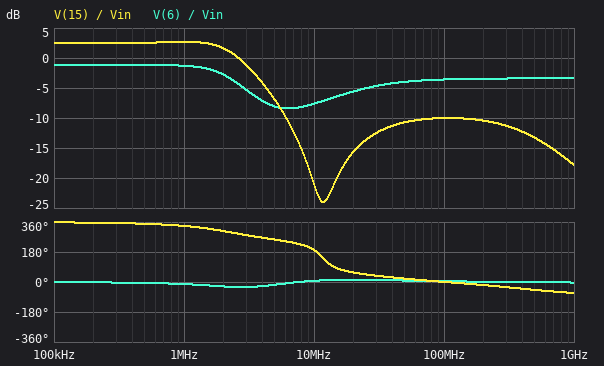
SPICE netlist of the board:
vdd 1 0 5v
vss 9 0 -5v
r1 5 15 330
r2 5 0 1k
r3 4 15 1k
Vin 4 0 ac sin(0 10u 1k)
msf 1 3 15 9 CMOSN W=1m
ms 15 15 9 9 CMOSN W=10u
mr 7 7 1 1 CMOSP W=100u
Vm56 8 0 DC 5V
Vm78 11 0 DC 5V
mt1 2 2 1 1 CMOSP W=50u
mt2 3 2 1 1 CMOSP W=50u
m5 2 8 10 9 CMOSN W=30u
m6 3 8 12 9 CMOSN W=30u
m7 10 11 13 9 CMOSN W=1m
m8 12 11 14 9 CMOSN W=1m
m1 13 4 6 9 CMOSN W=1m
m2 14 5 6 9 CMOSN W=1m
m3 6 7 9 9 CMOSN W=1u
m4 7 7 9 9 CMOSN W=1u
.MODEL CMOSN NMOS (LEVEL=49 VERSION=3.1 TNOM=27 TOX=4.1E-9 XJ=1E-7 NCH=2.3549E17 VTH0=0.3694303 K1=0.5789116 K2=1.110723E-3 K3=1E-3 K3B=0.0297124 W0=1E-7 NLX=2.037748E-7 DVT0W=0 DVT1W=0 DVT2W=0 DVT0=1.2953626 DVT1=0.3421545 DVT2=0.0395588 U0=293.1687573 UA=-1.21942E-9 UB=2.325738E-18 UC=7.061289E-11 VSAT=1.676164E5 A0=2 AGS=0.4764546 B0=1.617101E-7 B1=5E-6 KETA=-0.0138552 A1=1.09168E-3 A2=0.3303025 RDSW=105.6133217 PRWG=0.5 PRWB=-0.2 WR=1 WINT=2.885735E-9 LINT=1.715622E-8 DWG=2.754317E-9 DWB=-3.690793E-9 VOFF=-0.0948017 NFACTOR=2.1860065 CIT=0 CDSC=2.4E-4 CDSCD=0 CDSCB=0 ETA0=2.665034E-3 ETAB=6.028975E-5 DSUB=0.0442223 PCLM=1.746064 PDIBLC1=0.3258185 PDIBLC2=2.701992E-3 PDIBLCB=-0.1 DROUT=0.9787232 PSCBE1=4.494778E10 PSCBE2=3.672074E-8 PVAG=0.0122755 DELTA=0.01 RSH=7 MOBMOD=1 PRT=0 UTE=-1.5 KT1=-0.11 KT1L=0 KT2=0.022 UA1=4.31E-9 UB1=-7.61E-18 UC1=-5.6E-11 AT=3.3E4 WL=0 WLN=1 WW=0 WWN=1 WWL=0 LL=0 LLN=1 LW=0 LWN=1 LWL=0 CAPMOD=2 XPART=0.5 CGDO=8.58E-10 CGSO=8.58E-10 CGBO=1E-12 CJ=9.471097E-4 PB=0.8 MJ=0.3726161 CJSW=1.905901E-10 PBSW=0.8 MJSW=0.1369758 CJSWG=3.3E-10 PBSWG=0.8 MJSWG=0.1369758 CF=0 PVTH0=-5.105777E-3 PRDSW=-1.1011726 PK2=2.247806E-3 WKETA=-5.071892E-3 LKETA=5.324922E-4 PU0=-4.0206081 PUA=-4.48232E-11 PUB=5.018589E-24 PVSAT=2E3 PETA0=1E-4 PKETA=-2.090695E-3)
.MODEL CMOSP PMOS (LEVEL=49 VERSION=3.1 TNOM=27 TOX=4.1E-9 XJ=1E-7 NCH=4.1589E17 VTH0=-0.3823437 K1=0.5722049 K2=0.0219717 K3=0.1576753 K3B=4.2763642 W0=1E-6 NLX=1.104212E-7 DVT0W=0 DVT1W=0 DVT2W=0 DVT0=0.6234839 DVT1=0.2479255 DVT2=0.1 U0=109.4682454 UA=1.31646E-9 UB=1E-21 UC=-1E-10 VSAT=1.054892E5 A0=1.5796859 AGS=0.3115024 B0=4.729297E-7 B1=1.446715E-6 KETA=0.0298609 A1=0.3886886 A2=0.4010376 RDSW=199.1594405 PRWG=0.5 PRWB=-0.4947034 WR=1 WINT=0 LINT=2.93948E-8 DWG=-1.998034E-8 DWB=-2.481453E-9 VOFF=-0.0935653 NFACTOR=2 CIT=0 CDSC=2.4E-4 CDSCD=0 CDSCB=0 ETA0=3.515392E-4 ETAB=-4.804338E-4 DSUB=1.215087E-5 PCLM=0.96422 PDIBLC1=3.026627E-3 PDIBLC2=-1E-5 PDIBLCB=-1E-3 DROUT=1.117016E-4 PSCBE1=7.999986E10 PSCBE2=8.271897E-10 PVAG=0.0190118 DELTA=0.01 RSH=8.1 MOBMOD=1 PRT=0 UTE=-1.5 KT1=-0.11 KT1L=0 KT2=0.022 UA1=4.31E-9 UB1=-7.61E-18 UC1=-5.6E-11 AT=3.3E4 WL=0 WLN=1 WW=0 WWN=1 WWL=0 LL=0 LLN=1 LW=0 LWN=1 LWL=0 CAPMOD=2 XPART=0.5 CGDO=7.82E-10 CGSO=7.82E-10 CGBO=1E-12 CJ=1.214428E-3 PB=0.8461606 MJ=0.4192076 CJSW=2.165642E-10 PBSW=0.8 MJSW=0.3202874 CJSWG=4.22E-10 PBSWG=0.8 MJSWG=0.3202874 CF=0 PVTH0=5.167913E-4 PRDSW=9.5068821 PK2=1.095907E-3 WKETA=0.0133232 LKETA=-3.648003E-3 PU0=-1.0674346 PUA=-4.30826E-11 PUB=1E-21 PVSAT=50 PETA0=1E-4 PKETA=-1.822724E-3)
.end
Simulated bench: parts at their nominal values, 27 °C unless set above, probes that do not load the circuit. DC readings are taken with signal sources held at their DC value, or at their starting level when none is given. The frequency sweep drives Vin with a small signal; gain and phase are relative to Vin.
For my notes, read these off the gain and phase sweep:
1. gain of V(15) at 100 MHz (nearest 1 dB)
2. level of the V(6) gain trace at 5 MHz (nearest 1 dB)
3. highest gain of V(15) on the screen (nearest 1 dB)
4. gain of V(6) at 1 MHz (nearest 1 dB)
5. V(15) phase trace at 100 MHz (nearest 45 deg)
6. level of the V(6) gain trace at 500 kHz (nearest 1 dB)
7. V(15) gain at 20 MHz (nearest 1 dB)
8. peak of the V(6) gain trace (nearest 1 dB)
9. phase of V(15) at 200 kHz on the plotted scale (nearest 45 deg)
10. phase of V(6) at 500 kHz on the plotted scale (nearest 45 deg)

-10 dB
-8 dB
3 dB
-1 dB
0 deg
-1 dB
-16 dB
-1 dB
360 deg
0 deg
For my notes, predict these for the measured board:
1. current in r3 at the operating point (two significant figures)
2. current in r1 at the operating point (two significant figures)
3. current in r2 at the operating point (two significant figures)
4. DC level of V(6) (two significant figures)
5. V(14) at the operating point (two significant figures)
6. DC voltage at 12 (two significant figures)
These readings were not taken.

6.3 µA
4.7 µA
4.7 µA
-1.1 V
1.5 V
1.5 V
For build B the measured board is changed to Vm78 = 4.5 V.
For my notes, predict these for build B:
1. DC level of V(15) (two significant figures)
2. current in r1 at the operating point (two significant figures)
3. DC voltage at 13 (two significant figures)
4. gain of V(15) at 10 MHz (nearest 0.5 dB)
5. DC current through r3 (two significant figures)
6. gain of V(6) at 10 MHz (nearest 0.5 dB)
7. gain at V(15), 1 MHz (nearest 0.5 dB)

5.9 mV
4.4 µA
2.9 V
-4.0 dB
5.9 µA
-12.5 dB
2.0 dB
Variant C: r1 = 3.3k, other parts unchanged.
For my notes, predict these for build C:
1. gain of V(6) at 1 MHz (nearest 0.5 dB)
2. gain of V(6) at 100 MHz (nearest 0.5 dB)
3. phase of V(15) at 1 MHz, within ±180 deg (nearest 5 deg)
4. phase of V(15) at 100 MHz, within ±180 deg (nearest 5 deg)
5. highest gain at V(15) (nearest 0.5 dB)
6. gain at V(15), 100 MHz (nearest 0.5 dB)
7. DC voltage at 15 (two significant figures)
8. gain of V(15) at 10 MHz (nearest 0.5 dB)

-4.0 dB
-3.5 dB
-65 deg
-10 deg
12.5 dB
-13.5 dB
20 mV
-24.0 dB
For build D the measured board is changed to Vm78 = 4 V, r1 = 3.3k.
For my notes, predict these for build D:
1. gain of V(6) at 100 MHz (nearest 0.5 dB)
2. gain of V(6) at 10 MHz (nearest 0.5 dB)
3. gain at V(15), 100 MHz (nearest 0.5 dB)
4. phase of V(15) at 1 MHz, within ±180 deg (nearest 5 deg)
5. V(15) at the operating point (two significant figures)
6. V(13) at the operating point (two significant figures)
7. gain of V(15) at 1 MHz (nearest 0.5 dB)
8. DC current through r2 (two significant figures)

-3.5 dB
-6.0 dB
-15.0 dB
-50 deg
15 mV
2.5 V
9.0 dB
3.5 µA
